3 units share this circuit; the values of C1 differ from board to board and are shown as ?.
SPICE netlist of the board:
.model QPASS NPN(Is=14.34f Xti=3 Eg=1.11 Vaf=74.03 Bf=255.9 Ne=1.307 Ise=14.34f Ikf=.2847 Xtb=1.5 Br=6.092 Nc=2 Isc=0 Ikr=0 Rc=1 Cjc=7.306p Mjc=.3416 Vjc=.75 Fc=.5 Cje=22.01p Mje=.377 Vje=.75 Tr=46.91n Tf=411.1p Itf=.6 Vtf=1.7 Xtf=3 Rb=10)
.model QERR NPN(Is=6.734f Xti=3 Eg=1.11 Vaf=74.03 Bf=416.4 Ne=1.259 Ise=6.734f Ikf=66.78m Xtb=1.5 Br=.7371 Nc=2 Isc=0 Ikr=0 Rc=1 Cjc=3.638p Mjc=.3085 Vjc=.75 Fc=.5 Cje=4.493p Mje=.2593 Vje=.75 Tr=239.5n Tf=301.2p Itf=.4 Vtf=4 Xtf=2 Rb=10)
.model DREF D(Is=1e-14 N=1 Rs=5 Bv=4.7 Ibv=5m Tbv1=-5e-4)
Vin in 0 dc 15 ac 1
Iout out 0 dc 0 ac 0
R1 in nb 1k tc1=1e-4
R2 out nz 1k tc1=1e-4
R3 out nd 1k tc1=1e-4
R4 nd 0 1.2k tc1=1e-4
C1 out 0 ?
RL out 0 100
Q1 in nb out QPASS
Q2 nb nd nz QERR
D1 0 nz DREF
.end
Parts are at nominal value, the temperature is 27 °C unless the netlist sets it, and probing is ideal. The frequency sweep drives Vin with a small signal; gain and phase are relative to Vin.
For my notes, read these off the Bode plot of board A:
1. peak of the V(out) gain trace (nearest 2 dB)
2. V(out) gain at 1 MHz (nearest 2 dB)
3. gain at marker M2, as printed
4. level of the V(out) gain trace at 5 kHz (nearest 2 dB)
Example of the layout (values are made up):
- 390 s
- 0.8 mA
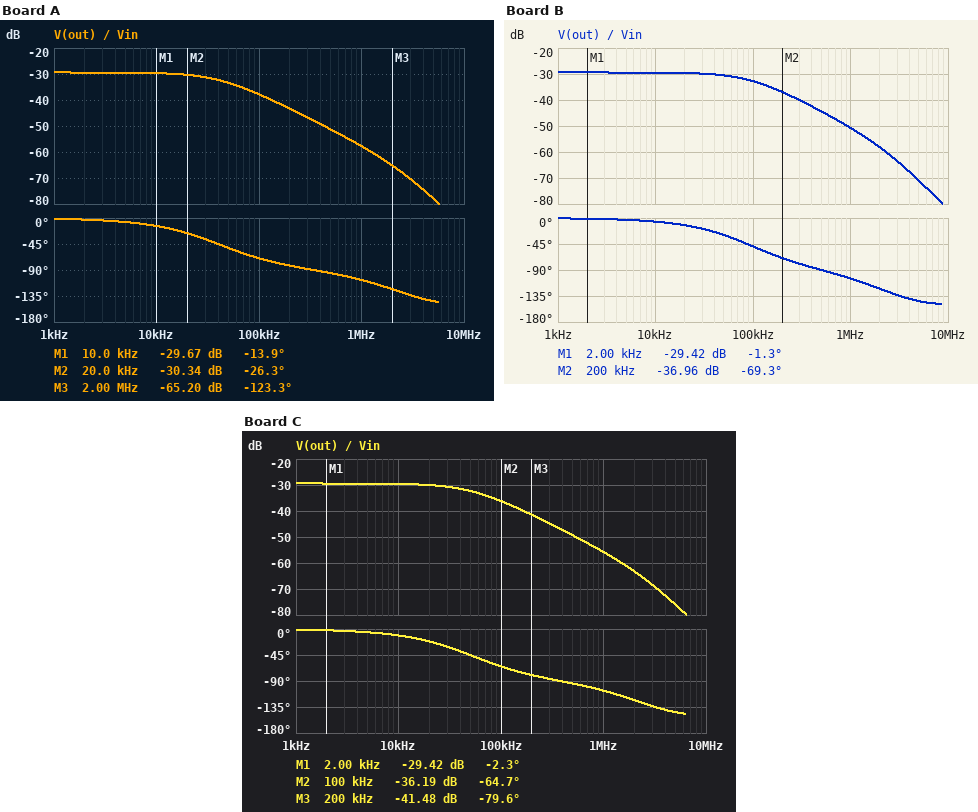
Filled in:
- -30 dB
- -58 dB
- -30.34 dB
- -30 dB
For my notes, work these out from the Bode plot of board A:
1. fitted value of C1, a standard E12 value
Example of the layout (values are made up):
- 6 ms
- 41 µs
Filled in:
- 15 µF
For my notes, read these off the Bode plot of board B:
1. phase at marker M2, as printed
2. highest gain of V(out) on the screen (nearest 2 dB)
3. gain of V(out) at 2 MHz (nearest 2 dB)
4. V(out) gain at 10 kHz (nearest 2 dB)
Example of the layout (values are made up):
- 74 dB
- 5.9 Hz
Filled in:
- -69.3 deg
- -30 dB
- -58 dB
- -30 dB
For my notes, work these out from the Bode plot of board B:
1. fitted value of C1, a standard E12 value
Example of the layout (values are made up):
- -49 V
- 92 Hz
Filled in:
- 6.8 µF
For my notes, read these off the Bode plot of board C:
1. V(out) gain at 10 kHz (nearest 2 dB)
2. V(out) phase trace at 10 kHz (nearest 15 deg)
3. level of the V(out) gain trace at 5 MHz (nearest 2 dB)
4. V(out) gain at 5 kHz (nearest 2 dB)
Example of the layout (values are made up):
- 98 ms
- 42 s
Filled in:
- -30 dB
- -15 deg
- -76 dB
- -30 dB
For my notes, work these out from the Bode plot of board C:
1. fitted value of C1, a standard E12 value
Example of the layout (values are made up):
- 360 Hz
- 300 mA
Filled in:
- 12 µF
